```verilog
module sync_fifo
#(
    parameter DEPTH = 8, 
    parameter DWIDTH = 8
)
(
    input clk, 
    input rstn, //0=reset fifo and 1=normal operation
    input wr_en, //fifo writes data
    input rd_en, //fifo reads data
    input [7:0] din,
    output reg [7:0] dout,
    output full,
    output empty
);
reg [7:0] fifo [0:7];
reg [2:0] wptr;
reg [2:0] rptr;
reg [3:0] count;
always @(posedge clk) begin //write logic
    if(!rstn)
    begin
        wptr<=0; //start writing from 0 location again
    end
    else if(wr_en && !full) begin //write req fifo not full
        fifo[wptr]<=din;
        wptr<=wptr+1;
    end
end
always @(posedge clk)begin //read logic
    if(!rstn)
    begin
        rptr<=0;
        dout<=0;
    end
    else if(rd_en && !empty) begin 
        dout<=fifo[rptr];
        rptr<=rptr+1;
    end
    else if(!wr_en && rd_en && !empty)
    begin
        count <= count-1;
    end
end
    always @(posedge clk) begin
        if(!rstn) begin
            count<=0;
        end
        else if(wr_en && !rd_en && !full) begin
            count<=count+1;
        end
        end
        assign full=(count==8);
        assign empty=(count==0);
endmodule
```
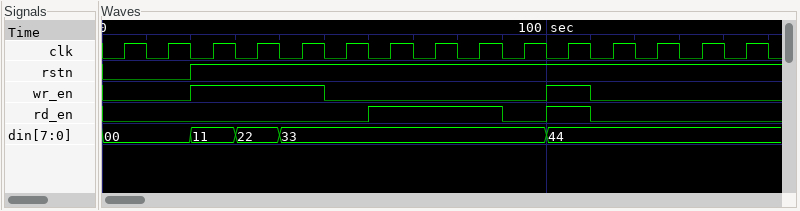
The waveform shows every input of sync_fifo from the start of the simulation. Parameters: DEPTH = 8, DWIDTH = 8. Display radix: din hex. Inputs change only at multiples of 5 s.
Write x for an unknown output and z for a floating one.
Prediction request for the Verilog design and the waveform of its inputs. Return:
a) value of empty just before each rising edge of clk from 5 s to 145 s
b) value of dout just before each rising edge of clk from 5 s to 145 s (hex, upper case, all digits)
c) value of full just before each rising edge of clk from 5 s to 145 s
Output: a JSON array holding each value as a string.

["x 1 1 0 0 0 0 0 0 0 0 0 0 0 0", "x, 00, 00, 00, 00, 00, 00, 11, 22, 33, 33, x, x, x, x", "x 0 0 0 0 0 0 0 0 0 0 0 0 0 0"]
